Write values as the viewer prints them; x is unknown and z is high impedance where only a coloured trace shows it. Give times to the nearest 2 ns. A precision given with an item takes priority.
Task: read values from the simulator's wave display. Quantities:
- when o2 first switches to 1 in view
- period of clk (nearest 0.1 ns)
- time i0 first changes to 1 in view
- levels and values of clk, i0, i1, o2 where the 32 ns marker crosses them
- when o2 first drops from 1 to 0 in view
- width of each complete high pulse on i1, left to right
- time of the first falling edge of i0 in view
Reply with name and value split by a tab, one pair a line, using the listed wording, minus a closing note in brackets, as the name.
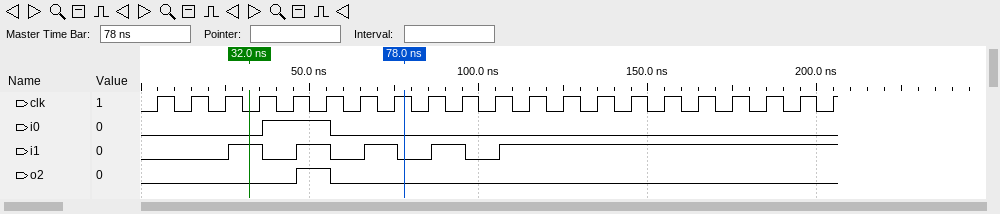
when o2 first switches to 1 in view	46 ns
period of clk	10 ns
time i0 first changes to 1 in view	36 ns
levels and values of clk, i0, i1, o2 where the 32 ns marker crosses them	clk=0, i0=0, i1=1, o2=0
when o2 first drops from 1 to 0 in view	56 ns
width of each complete high pulse on i1, left to right	10 ns, 10 ns, 10 ns, 10 ns
time of the first falling edge of i0 in view	56 ns
